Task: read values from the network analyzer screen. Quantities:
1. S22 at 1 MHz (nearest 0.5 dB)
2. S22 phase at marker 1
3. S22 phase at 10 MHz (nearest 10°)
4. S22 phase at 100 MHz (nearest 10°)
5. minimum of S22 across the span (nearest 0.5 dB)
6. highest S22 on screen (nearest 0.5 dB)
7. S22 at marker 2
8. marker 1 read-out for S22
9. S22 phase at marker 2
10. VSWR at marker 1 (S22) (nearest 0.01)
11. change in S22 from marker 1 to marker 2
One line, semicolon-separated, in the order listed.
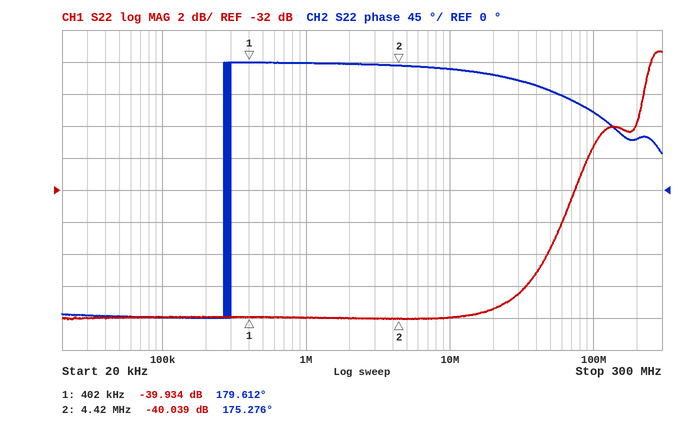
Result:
-40.0 dB; 179.612°; 170°; 110°; -40.0 dB; -23.5 dB; -40.039 dB; -39.934 dB; 175.276°; 1.02; -0.105 dB
